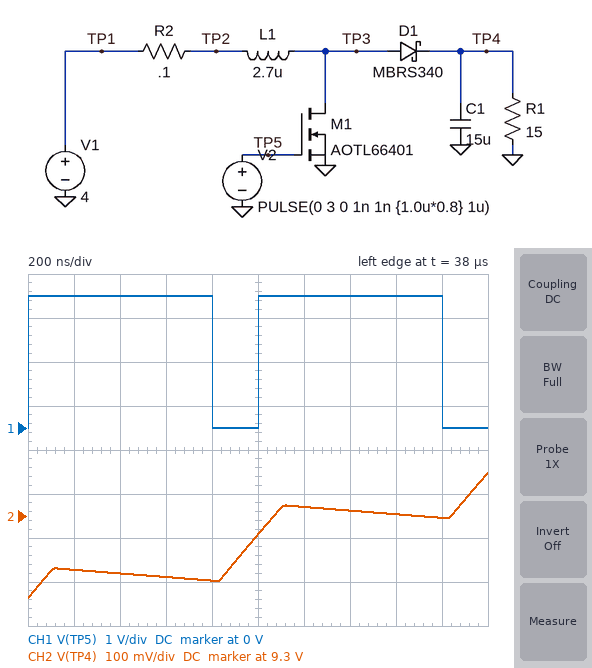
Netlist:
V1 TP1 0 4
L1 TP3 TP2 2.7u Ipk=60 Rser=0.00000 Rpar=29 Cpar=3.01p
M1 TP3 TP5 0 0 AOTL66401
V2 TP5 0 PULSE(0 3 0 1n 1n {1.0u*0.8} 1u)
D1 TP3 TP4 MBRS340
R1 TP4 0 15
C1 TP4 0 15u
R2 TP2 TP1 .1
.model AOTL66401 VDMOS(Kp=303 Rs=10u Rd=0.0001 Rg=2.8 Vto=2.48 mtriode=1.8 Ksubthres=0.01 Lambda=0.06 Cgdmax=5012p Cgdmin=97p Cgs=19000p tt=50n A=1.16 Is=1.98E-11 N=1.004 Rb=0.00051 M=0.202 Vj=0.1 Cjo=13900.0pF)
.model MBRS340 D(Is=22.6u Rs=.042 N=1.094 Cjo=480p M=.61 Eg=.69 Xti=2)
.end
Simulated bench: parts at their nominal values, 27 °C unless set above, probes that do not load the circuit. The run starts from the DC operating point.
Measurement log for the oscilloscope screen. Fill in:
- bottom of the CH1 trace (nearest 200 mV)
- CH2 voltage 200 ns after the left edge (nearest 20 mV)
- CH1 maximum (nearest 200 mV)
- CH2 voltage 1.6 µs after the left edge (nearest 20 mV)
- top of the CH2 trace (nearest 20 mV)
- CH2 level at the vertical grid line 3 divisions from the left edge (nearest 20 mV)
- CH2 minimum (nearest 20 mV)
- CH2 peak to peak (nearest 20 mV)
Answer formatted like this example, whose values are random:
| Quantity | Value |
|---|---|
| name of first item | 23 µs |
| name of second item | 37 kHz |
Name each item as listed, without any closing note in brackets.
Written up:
| Quantity | Value |
|---|---|
| bottom of the CH1 trace | 0 V |
| CH2 voltage 200 ns after the left edge | 9.18 V |
| CH1 maximum | 3.0 V |
| CH2 voltage 1.6 µs after the left edge | 9.30 V |
| top of the CH2 trace | 9.40 V |
| CH2 level at the vertical grid line 3 divisions from the left edge | 9.16 V |
| CH2 minimum | 9.12 V |
| CH2 peak to peak | 280 mV |
